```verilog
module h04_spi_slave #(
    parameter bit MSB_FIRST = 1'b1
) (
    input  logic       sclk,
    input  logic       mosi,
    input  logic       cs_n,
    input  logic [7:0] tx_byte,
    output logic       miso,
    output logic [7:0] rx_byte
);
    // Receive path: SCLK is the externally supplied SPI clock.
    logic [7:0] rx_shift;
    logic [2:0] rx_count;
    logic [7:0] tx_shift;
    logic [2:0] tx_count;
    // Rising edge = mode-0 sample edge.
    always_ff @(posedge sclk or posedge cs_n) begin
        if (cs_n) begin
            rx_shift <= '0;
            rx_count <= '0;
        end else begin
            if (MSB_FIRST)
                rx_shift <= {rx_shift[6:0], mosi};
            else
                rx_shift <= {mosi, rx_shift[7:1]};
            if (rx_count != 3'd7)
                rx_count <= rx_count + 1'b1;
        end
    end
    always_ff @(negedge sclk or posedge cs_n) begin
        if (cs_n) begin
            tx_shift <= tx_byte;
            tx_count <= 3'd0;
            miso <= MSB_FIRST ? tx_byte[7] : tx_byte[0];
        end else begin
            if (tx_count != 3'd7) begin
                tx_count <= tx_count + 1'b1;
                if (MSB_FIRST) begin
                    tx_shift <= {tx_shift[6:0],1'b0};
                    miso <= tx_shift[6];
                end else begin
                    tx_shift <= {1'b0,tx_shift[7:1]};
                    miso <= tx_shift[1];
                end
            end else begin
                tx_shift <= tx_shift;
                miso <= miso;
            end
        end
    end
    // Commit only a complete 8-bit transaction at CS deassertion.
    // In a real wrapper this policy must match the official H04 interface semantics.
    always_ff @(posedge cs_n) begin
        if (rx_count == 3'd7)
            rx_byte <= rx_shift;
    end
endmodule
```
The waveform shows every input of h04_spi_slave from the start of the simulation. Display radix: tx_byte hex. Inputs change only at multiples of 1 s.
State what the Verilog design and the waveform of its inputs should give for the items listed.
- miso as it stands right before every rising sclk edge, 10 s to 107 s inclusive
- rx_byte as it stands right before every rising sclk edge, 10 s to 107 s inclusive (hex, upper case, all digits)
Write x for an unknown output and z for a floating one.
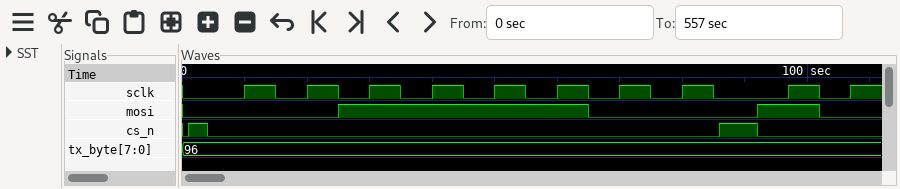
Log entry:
1 0 0 1 0 1 1 0 1 0
x, x, x, x, x, x, x, x, 3C, 3C
